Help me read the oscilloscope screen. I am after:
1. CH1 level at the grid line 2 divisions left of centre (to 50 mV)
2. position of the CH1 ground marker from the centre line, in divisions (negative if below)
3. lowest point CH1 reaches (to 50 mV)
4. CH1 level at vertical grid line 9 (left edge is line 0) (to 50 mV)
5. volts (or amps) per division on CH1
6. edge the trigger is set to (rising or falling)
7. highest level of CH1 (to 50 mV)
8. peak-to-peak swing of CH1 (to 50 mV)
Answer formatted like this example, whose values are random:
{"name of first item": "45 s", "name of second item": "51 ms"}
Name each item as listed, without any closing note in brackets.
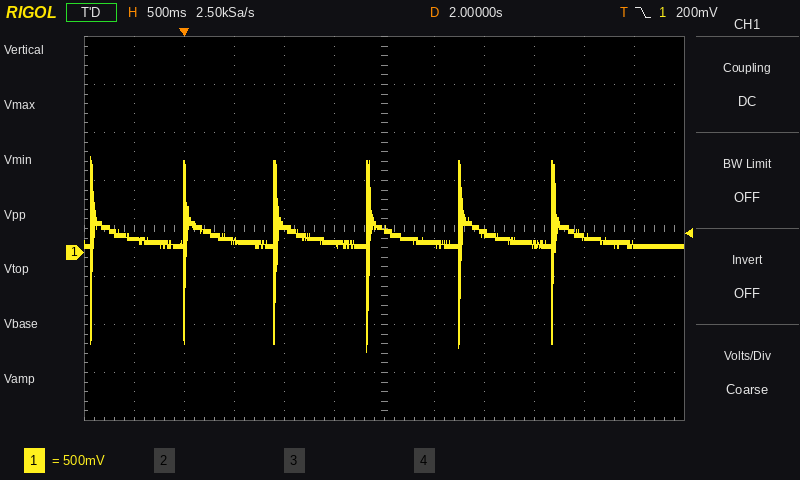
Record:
{"CH1 level at the grid line 2 divisions left of centre": "300 mV", "position of the CH1 ground marker from the centre line, in divisions": "-0.5 div", "lowest point CH1 reaches": "-1.05 V", "CH1 level at vertical grid line 9 (left edge is line 0)": "100 mV", "volts (or amps) per division on CH1": "500 mV", "edge the trigger is set to": "falling", "highest level of CH1": "1.00 V", "peak-to-peak swing of CH1": "2.05 V"}
